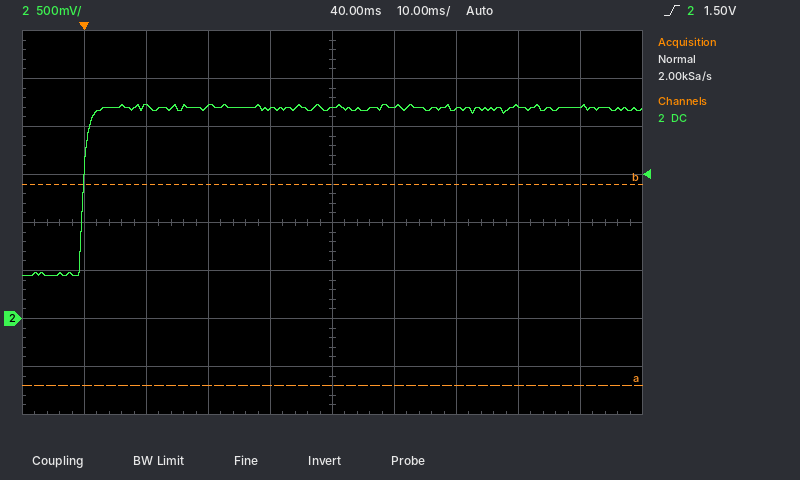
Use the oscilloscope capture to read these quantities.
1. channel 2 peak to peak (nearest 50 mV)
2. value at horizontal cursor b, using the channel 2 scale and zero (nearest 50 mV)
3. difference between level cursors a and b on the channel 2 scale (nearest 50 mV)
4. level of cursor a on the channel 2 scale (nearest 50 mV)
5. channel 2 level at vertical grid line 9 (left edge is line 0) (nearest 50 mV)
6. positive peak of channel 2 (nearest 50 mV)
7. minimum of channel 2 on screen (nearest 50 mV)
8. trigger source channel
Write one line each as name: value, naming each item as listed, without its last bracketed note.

channel 2 peak to peak: 1.80 V
value at horizontal cursor b, using the channel 2 scale and zero: 1.40 V
difference between level cursors a and b on the channel 2 scale: 2.10 V
level of cursor a on the channel 2 scale: -700 mV
channel 2 level at vertical grid line 9 (left edge is line 0): 2.20 V
positive peak of channel 2: 2.25 V
minimum of channel 2 on screen: 450 mV
trigger source channel: channel 2
